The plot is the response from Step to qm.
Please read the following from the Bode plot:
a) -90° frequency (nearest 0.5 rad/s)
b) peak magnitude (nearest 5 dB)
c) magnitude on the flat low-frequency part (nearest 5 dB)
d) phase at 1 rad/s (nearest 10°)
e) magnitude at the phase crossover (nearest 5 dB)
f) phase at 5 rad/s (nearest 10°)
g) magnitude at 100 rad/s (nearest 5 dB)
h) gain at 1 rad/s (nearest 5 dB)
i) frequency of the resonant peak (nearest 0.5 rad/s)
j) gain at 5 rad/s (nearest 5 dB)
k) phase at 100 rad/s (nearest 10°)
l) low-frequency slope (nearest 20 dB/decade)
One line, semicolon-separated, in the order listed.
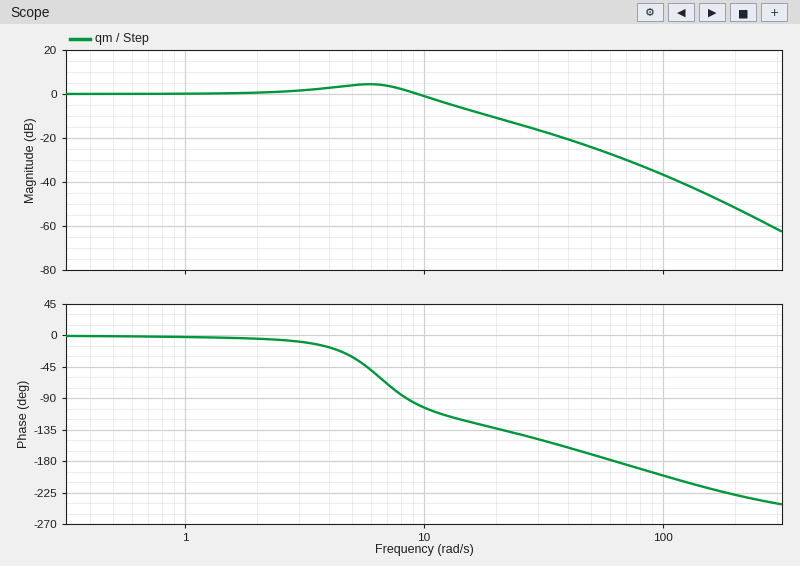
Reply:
8.5 rad/s; 5 dB; 0 dB; 0°; -30 dB; -30°; -35 dB; 0 dB; 6.0 rad/s; 5 dB; -200°; 0 dB/decade
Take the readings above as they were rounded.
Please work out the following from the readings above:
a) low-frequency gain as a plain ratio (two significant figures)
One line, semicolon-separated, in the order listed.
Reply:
1.0
